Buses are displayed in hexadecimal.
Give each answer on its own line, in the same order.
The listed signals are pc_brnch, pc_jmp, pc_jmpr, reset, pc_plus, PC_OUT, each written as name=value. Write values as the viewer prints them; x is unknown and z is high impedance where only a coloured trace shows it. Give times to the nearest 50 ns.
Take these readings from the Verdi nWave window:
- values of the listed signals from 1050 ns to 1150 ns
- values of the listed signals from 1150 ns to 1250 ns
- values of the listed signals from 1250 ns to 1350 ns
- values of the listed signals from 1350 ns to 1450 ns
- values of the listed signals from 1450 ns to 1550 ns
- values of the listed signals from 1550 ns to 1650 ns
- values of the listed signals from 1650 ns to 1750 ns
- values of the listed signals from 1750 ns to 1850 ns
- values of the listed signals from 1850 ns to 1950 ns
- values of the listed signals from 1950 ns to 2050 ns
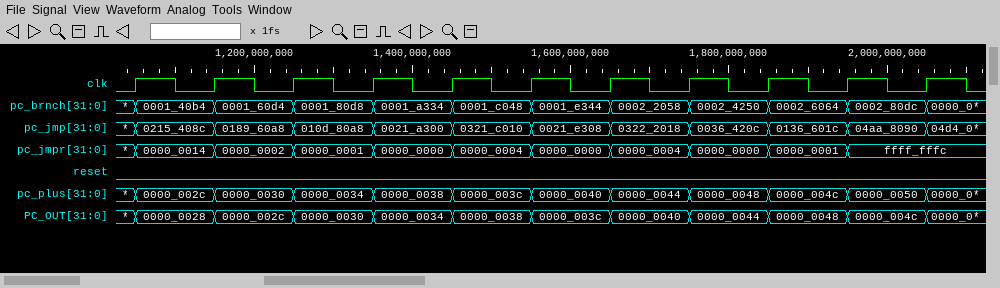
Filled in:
pc_brnch=0001_40b4, pc_jmp=0215_408c, pc_jmpr=0000_0014, reset=0, pc_plus=0000_002c, PC_OUT=0000_0028
pc_brnch=0001_60d4, pc_jmp=0189_60a8, pc_jmpr=0000_0002, reset=0, pc_plus=0000_0030, PC_OUT=0000_002c
pc_brnch=0001_80d8, pc_jmp=010d_80a8, pc_jmpr=0000_0001, reset=0, pc_plus=0000_0034, PC_OUT=0000_0030
pc_brnch=0001_a334, pc_jmp=0021_a300, pc_jmpr=0000_0000, reset=0, pc_plus=0000_0038, PC_OUT=0000_0034
pc_brnch=0001_c048, pc_jmp=0321_c010, pc_jmpr=0000_0004, reset=0, pc_plus=0000_003c, PC_OUT=0000_0038
pc_brnch=0001_e344, pc_jmp=0021_e308, pc_jmpr=0000_0000, reset=0, pc_plus=0000_0040, PC_OUT=0000_003c
pc_brnch=0002_2058, pc_jmp=0322_2018, pc_jmpr=0000_0004, reset=0, pc_plus=0000_0044, PC_OUT=0000_0040
pc_brnch=0002_4250, pc_jmp=0036_420c, pc_jmpr=0000_0000, reset=0, pc_plus=0000_0048, PC_OUT=0000_0044
pc_brnch=0002_6064, pc_jmp=0136_601c, pc_jmpr=0000_0001, reset=0, pc_plus=0000_004c, PC_OUT=0000_0048
pc_brnch=0002_80dc, pc_jmp=04aa_8090, pc_jmpr=ffff_fffc, reset=0, pc_plus=0000_0050, PC_OUT=0000_004c
